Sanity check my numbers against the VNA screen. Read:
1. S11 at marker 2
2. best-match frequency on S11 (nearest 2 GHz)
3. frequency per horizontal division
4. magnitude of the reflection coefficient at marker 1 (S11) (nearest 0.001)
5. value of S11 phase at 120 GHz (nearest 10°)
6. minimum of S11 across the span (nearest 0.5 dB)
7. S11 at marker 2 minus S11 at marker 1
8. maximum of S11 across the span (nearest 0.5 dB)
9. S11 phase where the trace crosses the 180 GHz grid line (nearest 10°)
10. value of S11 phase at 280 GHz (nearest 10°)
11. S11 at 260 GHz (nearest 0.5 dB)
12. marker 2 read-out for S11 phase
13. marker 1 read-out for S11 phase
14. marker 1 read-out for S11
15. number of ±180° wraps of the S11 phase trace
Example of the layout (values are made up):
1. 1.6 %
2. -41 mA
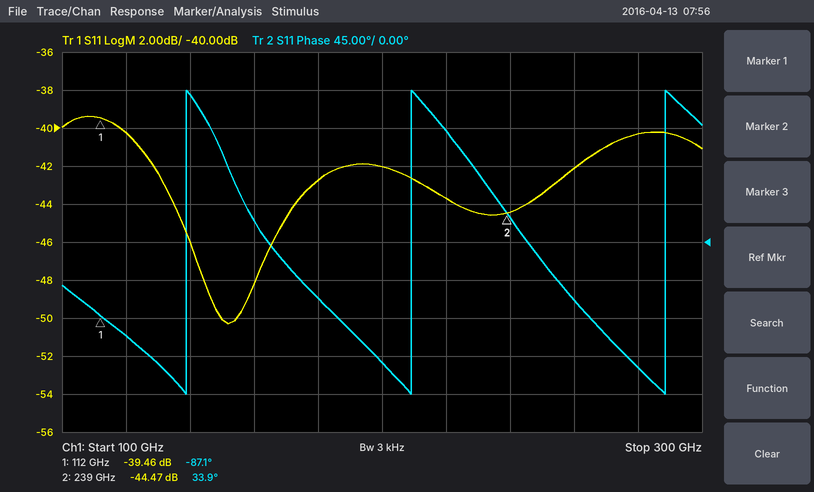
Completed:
1. -44.47 dB
2. 152 GHz
3. 20 GHz
4. 0.011
5. -110°
6. -50.5 dB
7. -5.01 dB
8. -39.5 dB
9. -70°
10. -150°
11. -42.0 dB
12. 33.9°
13. -87.1°
14. -39.46 dB
15. 3
